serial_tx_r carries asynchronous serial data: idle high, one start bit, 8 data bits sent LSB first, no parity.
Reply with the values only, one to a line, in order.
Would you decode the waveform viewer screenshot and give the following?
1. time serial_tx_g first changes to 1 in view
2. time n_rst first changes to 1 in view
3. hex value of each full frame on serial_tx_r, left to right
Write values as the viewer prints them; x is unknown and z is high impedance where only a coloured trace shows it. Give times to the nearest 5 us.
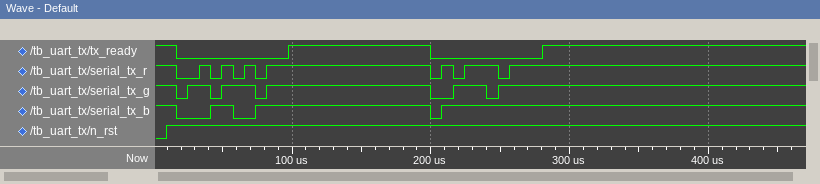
25 us
10 us
AA, DD
